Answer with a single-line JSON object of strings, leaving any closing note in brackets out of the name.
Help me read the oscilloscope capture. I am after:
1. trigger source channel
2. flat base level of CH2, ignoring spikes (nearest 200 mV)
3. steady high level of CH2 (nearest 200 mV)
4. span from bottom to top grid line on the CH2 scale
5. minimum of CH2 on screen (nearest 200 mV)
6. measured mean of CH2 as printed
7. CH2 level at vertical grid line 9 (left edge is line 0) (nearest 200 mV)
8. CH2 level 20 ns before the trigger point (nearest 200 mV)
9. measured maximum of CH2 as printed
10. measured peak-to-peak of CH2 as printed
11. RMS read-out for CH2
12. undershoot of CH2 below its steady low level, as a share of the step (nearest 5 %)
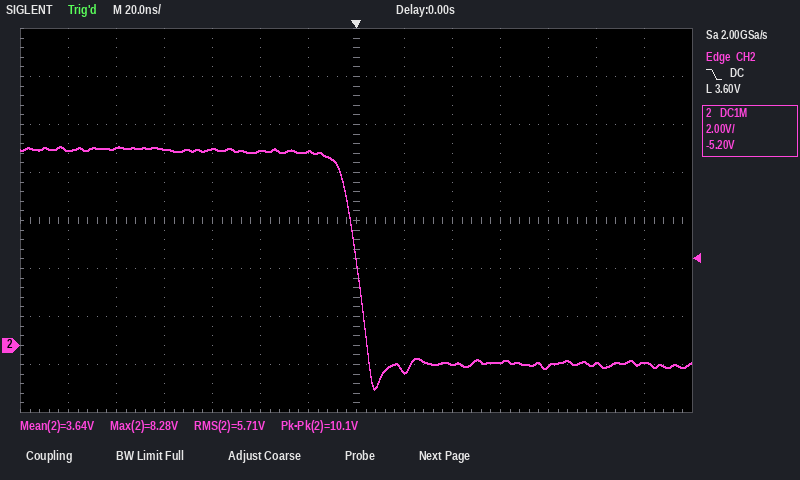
{"trigger source channel": "CH2", "flat base level of CH2, ignoring spikes": "-800 mV", "steady high level of CH2": "8.2 V", "span from bottom to top grid line on the CH2 scale": "16 V", "minimum of CH2 on screen": "-1.8 V", "measured mean of CH2 as printed": "3.64 V", "CH2 level at vertical grid line 9 (left edge is line 0)": "-800 mV", "CH2 level 20 ns before the trigger point": "8.0 V", "measured maximum of CH2 as printed": "8.28 V", "measured peak-to-peak of CH2 as printed": "10.1 V", "RMS read-out for CH2": "5.71 V", "undershoot of CH2 below its steady low level, as a share of the step": "10 %"}
